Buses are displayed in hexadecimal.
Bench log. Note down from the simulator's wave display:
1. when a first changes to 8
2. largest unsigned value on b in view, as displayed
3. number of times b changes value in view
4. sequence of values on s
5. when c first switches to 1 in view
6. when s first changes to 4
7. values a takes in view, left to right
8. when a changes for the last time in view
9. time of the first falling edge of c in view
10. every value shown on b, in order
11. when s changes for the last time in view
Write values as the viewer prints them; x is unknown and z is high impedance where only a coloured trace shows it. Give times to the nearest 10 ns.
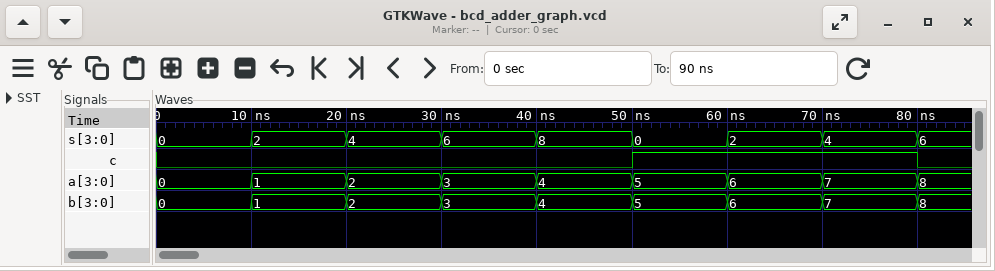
80 ns
8
8
0, 2, 4, 6, 8, 0, 2, 4, 6
50 ns
20 ns
0, 1, 2, 3, 4, 5, 6, 7, 8
80 ns
80 ns
0, 1, 2, 3, 4, 5, 6, 7, 8
80 ns
